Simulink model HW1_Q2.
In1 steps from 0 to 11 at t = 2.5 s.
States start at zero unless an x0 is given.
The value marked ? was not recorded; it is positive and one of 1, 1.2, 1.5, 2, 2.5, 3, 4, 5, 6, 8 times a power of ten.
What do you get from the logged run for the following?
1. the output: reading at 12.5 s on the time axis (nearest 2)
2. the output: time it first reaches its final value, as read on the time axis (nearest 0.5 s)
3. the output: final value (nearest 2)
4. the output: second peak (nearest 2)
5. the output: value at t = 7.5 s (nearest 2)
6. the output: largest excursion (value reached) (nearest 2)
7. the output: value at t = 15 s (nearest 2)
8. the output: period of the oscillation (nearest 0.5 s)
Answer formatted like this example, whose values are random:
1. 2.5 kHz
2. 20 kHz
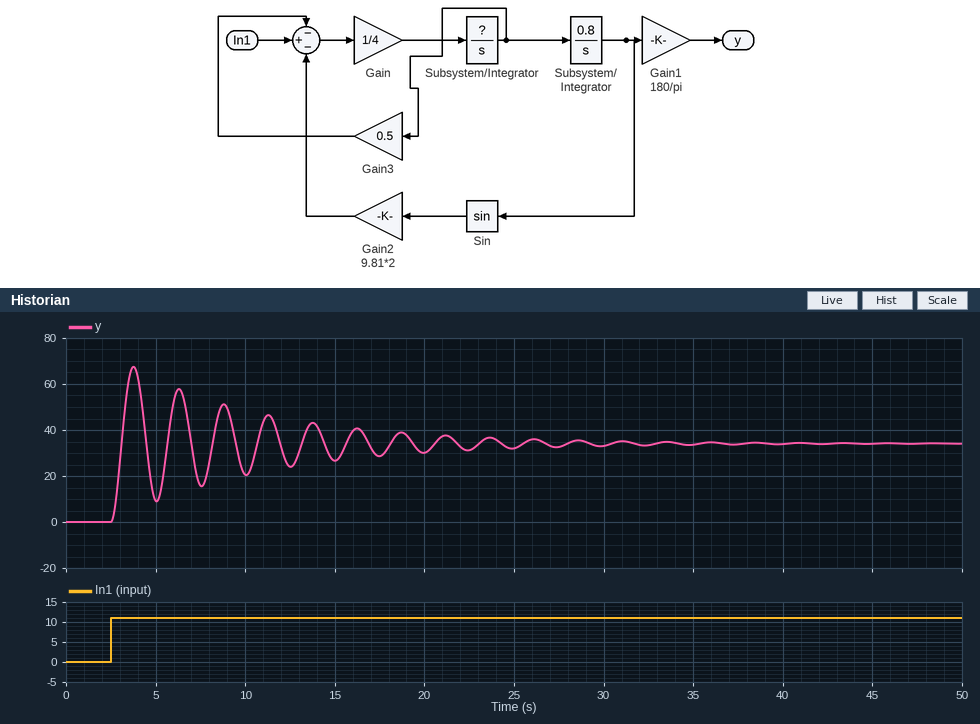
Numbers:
1. 24
2. 3.0 s
3. 34
4. 58
5. 16
6. 68
7. 26
8. 2.5 s
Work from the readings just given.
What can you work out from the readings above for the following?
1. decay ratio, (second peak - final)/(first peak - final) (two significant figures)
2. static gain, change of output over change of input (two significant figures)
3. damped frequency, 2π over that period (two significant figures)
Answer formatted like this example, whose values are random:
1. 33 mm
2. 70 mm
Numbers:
1. 0.71
2. 3.1
3. 2.5 rad/s
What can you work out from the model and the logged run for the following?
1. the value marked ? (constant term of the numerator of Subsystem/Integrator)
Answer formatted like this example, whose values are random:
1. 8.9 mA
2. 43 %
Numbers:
1. 2
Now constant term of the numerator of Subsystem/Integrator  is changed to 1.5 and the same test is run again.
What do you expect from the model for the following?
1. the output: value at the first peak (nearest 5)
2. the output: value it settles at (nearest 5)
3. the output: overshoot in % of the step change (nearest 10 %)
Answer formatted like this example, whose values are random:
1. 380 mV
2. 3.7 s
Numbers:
1. 70
2. 35
3. 100 %
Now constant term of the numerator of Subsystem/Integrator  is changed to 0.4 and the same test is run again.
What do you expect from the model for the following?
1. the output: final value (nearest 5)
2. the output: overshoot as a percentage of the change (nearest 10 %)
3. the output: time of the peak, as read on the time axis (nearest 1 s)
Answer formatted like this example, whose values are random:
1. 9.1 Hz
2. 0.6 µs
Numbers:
1. 35
2. 90 %
3. 4 s
